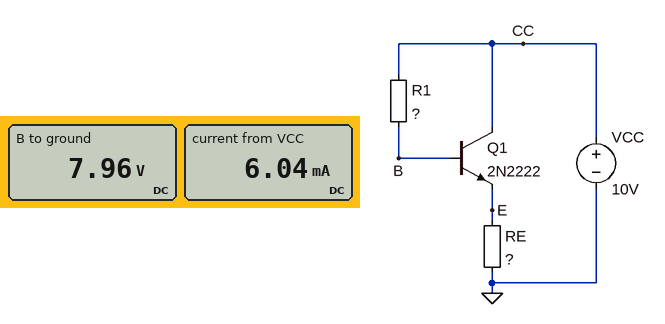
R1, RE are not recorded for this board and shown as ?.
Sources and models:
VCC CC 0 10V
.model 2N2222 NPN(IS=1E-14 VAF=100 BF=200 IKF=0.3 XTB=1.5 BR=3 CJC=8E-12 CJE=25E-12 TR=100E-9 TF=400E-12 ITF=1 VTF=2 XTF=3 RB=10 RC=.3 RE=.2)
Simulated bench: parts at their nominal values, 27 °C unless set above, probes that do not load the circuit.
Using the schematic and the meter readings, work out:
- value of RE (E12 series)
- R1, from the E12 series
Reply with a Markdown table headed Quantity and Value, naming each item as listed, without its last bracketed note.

| Quantity | Value |
|---|---|
| value of RE | 1.2 kΩ |
| R1, from the E12 series | 68 kΩ |
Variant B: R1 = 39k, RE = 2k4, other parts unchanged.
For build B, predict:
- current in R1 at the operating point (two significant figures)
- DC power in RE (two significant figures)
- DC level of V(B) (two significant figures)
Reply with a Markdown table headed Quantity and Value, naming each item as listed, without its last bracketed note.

| Quantity | Value |
|---|---|
| current in R1 at the operating point | 18 µA |
| DC power in RE | 31 mW |
| DC level of V(B) | 9.3 V |
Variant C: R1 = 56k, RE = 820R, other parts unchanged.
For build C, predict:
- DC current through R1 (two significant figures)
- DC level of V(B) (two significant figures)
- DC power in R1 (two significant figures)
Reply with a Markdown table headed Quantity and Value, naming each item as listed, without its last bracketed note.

| Quantity | Value |
|---|---|
| DC current through R1 | 42 µA |
| DC level of V(B) | 7.6 V |
| DC power in R1 | 100 µW |
